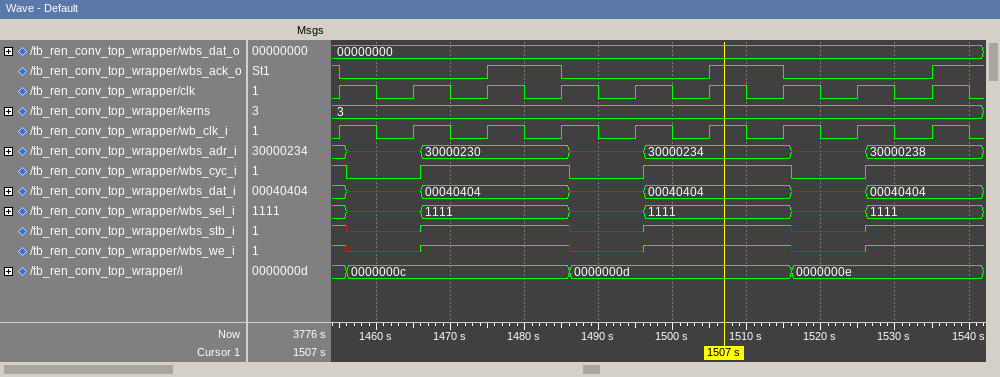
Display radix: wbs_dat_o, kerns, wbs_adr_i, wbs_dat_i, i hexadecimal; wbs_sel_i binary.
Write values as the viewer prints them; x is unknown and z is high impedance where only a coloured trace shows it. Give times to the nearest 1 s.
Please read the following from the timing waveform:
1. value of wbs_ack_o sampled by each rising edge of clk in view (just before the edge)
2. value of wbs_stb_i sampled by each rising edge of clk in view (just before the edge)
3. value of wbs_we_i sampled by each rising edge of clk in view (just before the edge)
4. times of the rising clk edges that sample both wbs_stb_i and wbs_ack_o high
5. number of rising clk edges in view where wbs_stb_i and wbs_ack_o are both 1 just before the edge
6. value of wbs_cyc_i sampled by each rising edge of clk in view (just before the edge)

1 0 0 1 0 0 1 0 0
1 x 1 1 x 1 1 x 1
1 x 1 1 x 1 1 x 1
1455 s, 1485 s, 1515 s
3
1 0 1 1 0 1 1 0 1
